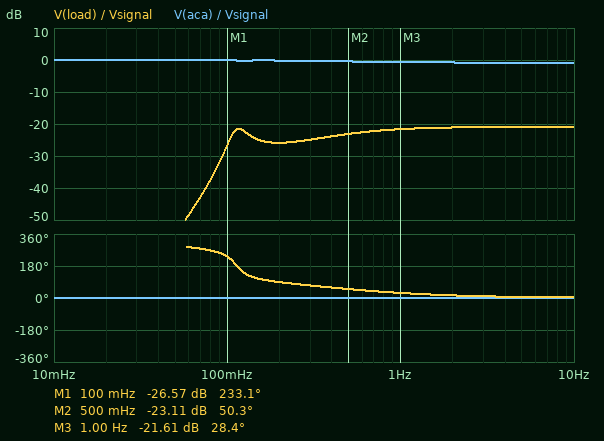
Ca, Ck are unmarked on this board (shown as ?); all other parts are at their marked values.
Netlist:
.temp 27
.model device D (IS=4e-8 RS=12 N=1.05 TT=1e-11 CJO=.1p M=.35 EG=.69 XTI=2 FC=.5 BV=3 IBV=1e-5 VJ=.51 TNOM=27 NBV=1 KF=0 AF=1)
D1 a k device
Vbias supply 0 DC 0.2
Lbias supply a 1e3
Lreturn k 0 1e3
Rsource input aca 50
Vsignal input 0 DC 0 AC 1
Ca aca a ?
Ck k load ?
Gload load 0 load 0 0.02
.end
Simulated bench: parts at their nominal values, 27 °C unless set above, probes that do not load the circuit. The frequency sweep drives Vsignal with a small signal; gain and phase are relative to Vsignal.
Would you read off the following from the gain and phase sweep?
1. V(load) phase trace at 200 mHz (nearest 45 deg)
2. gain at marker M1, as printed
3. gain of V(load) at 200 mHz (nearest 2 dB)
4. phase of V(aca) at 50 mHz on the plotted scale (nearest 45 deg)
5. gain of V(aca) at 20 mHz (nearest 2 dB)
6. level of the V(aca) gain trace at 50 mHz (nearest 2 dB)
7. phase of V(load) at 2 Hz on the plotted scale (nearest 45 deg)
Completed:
90 deg
-26.57 dB
-26 dB
0 deg
0 dB
0 dB
0 deg
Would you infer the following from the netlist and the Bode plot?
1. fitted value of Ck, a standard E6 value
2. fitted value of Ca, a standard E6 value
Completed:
3.3 mF
680 µF
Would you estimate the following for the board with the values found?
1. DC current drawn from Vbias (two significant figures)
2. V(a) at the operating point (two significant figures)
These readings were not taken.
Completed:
61 µA
200 mV
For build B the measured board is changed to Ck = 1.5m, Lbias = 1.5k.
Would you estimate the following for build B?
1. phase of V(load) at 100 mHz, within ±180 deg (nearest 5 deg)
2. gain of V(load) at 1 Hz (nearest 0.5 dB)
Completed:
-90 deg
-22.0 dB
